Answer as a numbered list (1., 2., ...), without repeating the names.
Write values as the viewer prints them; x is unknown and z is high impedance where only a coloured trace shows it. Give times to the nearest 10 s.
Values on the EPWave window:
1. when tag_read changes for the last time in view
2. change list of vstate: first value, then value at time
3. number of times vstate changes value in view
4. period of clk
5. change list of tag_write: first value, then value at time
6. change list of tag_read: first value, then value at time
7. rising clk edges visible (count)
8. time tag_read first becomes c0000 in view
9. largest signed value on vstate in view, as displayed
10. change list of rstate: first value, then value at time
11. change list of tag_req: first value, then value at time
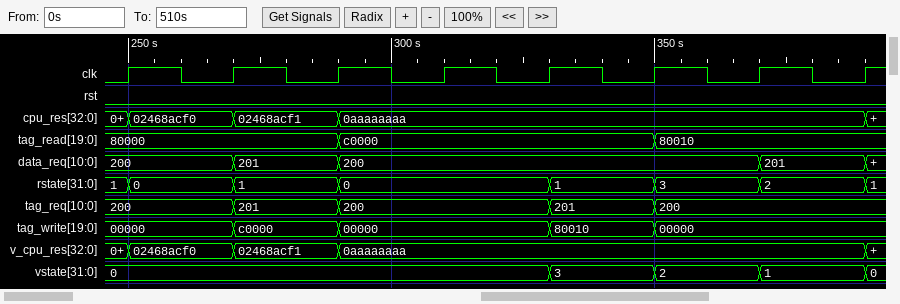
1. 350 s
2. 0, 3 at 330 s, 2 at 350 s, 1 at 370 s, 0 at 390 s
3. 4
4. 20 s
5. 00000, c0000 at 270 s, 00000 at 290 s, 80010 at 330 s, 00000 at 350 s
6. 80000, c0000 at 290 s, 80010 at 350 s
7. 8
8. 290 s
9. 3
10. 1, 0 at 250 s, 1 at 270 s, 0 at 290 s, 1 at 330 s, 3 at 350 s, 2 at 370 s, 1 at 390 s
11. 200, 201 at 270 s, 200 at 290 s, 201 at 330 s, 200 at 350 s
